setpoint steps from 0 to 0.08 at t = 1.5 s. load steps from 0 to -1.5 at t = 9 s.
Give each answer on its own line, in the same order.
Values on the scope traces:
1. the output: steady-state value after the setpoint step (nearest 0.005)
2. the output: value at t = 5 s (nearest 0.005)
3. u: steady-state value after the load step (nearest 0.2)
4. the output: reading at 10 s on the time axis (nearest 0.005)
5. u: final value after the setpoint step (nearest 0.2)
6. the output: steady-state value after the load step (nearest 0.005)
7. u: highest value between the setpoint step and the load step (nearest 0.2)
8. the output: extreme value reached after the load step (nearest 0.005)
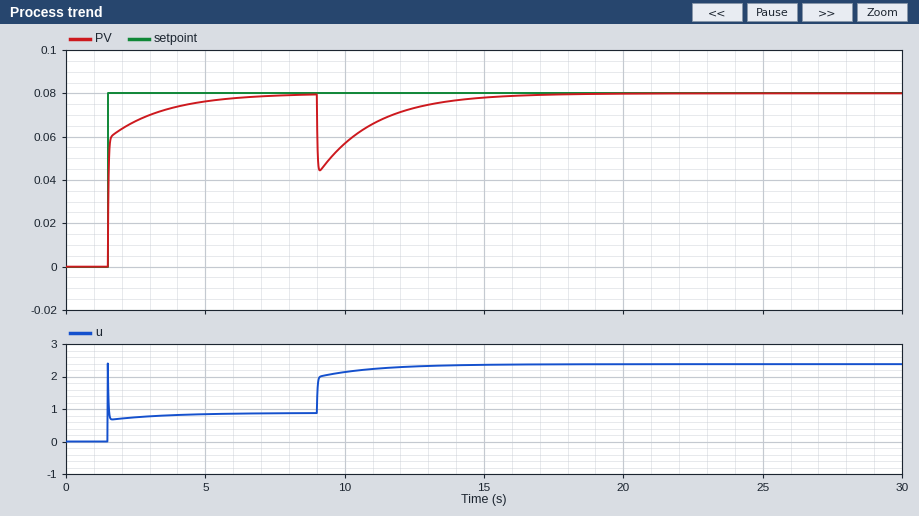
0.080
0.075
2.4
0.055
0.8
0.080
2.4
0.045
